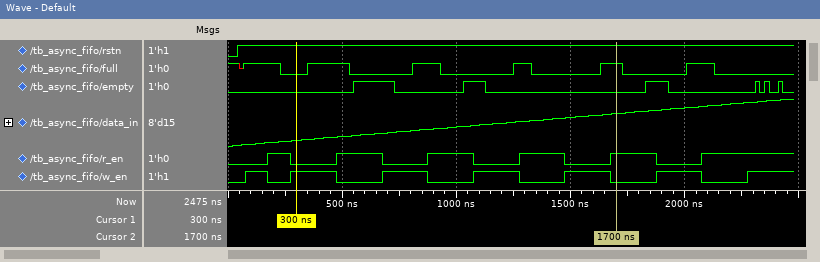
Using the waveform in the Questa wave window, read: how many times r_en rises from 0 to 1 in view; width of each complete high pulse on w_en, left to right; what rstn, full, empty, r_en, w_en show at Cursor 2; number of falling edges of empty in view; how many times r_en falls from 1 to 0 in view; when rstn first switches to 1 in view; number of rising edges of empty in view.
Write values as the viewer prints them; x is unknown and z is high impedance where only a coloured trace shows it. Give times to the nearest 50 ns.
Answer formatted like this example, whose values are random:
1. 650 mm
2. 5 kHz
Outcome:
1. 6
2. 100 ns, 200 ns, 200 ns, 200 ns, 200 ns, 200 ns
3. rstn=1, full=1, empty=0, r_en=1, w_en=0
4. 6
5. 5
6. 50 ns
7. 6
